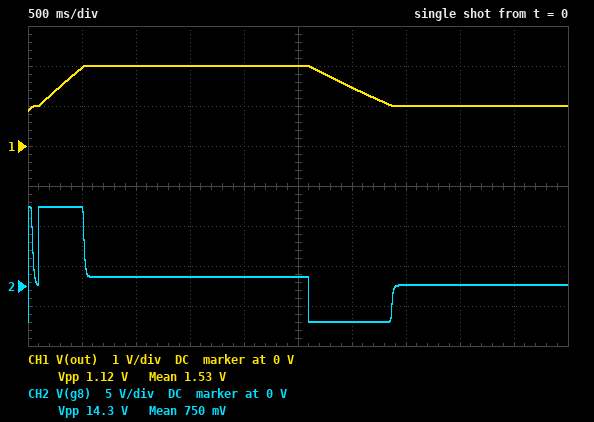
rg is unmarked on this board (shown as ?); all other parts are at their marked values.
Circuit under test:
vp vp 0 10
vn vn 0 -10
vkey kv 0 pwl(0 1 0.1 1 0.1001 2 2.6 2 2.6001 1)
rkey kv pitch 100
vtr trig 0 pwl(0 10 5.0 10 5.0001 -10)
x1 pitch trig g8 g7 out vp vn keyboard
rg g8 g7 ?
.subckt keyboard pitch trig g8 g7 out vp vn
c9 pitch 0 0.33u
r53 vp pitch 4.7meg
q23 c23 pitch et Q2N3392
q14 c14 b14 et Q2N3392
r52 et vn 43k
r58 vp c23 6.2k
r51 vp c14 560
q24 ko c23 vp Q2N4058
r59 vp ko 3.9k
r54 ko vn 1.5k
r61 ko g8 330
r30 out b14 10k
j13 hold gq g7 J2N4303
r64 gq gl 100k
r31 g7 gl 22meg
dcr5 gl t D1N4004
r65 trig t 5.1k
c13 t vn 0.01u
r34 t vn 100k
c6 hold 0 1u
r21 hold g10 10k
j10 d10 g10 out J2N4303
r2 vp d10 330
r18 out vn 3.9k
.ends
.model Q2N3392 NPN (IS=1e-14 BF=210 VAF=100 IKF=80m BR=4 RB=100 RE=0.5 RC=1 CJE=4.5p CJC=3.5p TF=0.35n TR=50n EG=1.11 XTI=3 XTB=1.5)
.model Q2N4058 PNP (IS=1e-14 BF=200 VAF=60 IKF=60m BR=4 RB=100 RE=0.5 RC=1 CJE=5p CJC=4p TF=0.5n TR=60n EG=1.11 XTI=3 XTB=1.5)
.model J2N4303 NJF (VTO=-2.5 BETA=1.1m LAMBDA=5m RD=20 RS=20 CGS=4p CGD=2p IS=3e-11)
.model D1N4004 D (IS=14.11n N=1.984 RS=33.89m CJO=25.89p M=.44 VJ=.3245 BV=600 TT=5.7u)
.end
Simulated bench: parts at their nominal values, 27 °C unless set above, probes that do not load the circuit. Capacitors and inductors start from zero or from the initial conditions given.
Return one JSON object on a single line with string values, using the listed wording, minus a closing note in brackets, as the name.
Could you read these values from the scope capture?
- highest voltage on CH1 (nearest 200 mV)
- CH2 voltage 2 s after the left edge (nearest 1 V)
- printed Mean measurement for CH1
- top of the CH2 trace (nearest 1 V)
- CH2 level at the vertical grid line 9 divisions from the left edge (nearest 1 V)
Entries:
{"highest voltage on CH1": "2.0 V", "CH2 voltage 2 s after the left edge": "1 V", "printed Mean measurement for CH1": "1.53 V", "top of the CH2 trace": "10 V", "CH2 level at the vertical grid line 9 divisions from the left edge": "0 V"}
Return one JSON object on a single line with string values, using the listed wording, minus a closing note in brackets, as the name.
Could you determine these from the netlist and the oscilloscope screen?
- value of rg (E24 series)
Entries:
{"value of rg": "3.6 MΩ"}
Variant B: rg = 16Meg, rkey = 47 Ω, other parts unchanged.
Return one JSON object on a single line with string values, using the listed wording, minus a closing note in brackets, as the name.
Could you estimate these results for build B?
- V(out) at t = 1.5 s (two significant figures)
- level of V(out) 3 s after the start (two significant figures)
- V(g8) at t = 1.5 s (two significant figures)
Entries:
{"V(out) at t = 1.5 s": "1.7 V", "level of V(out) 3 s after the start": "1.9 V", "V(g8) at t = 1.5 s": "9.9 V"}
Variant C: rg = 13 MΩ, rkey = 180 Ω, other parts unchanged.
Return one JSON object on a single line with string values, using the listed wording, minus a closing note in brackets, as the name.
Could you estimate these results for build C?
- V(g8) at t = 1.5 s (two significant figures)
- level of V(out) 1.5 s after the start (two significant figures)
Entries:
{"V(g8) at t = 1.5 s": "9.9 V", "level of V(out) 1.5 s after the start": "1.9 V"}
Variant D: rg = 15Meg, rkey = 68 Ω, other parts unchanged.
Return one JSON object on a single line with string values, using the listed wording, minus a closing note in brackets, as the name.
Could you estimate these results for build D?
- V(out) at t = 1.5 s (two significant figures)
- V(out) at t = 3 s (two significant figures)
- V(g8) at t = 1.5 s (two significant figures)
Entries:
{"V(out) at t = 1.5 s": "1.8 V", "V(out) at t = 3 s": "1.9 V", "V(g8) at t = 1.5 s": "9.9 V"}
